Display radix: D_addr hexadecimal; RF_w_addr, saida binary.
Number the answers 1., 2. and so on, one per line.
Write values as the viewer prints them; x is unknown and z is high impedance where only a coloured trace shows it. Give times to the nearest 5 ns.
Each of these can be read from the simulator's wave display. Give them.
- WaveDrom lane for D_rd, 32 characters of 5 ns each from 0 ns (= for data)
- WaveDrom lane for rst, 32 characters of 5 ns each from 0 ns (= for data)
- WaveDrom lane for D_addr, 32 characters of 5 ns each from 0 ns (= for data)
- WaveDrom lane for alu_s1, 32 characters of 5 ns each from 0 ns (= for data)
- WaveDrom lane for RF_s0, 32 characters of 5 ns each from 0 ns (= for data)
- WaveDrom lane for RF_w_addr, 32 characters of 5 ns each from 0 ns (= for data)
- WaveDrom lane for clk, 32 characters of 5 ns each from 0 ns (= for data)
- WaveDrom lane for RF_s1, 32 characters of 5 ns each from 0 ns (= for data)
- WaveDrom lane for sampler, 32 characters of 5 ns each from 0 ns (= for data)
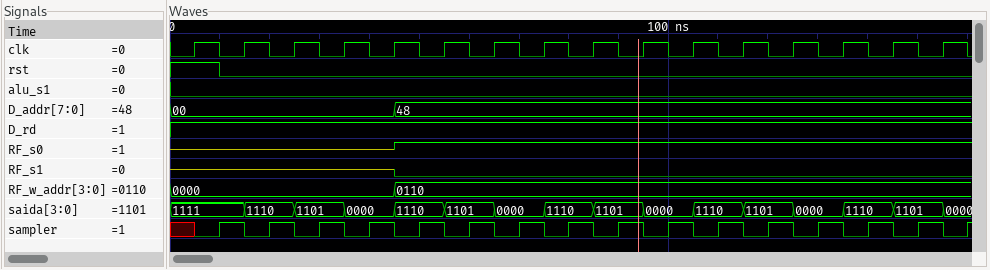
1. {name: 'D_rd', wave: '1...............................'}
2. {name: 'rst', wave: '1.0.............................'}
3. {name: 'D_addr', wave: '=........=......................', data: '00 48'}
4. {name: 'alu_s1', wave: '0...............................'}
5. {name: 'RF_s0', wave: 'z........1......................'}
6. {name: 'RF_w_addr', wave: '=........=......................', data: '0000 0110'}
7. {name: 'clk', wave: '01010101010101010101010101010101'}
8. {name: 'RF_s1', wave: 'z........0......................'}
9. {name: 'sampler', wave: 'x0101010101010101010101010101010'}
